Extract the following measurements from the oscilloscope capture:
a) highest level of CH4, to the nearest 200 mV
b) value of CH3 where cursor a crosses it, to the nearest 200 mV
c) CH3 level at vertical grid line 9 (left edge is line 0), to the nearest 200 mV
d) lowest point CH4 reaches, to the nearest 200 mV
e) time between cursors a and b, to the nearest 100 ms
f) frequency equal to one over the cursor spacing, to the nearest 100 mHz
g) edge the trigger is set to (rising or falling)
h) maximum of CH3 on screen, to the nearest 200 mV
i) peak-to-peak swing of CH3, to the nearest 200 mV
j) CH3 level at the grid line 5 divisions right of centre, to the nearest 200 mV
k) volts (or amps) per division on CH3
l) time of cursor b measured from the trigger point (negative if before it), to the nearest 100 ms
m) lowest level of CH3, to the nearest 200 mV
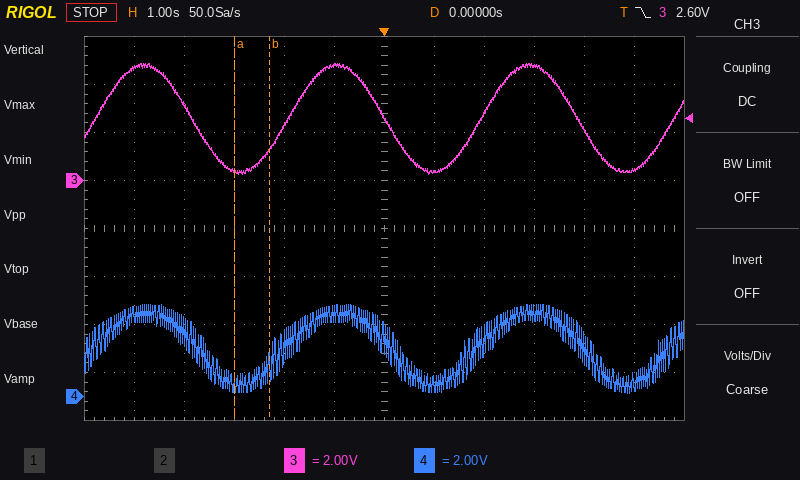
3.8 V
400 mV
4.8 V
200 mV
700 ms
1.4 Hz
falling
4.8 V
4.6 V
400 mV
2 V
-2.3 s
200 mV
